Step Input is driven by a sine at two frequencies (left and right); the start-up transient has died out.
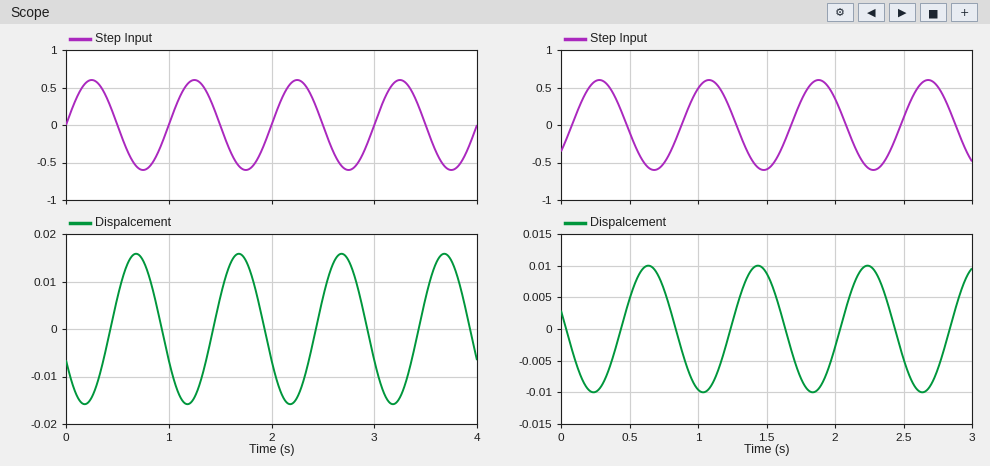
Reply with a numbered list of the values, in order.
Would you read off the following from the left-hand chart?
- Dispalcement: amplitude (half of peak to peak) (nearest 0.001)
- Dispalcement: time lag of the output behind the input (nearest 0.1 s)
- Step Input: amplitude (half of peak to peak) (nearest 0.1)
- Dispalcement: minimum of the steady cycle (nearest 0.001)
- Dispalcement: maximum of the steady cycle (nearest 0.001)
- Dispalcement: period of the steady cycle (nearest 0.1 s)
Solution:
1. 0.016
2. 0.4 s
3. 0.6
4. -0.016
5. 0.016
6. 1.0 s
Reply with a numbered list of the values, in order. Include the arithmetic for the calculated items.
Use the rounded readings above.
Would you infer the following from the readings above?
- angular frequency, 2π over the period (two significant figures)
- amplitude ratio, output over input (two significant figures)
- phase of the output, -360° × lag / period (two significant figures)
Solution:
1. 2π / 1 = 6.3 rad/s
2. 0.016 / 0.6 = 0.027
3. -360 × 0.4 / 1 = -140°
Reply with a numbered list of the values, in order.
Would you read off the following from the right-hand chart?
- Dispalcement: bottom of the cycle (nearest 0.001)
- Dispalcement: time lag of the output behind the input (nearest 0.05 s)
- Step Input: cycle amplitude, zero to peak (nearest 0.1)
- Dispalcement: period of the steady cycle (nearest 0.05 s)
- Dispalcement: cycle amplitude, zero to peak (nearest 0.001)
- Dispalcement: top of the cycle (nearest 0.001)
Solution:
1. -0.010
2. 0.35 s
3. 0.6
4. 0.80 s
5. 0.010
6. 0.010
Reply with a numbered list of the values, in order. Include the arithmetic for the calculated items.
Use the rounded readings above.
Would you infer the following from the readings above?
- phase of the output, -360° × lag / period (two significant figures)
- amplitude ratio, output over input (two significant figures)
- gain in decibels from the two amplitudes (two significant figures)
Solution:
1. -360 × 0.35 / 0.8 = -160°
2. 0.01 / 0.6 = 0.017
3. 20 log10(0.01 / 0.6) = -36 dB
